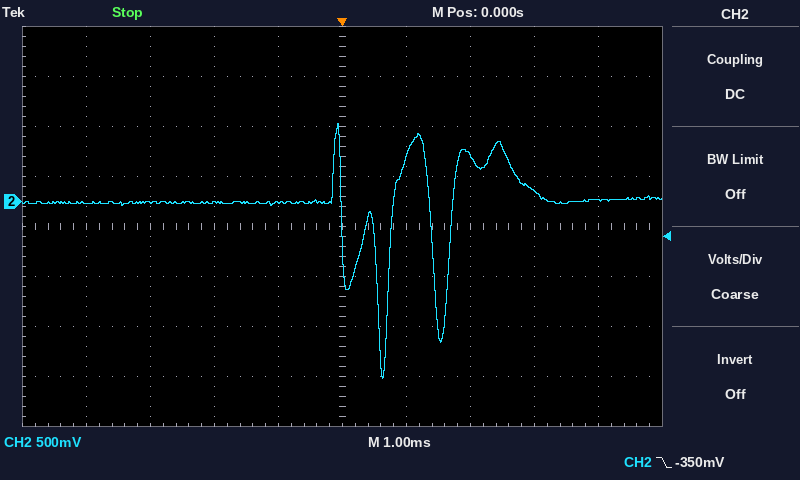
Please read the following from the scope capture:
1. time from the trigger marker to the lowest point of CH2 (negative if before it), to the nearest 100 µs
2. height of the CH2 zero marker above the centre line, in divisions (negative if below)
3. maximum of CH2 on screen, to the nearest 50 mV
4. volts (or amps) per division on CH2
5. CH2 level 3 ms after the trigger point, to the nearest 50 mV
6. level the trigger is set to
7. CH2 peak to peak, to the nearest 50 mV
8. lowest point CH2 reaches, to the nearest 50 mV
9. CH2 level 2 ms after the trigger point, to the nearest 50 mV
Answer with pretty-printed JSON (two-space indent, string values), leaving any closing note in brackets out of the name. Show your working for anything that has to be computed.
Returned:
{
  "time from the trigger marker to the lowest point of CH2 (negative if before it), to the nearest 100 µs": "+600 µs",
  "height of the CH2 zero marker above the centre line, in divisions": "+0.5 div",
  "maximum of CH2 on screen, to the nearest 50 mV": "800 mV",
  "volts (or amps) per division on CH2": "500 mV",
  "CH2 level 3 ms after the trigger point, to the nearest 50 mV": "100 mV",
  "level the trigger is set to": "-350 mV",
  "CH2 peak to peak, to the nearest 50 mV": "800 mV − (-1.75 V) = 2.55 V",
  "lowest point CH2 reaches, to the nearest 50 mV": "-1.75 V",
  "CH2 level 2 ms after the trigger point, to the nearest 50 mV": "450 mV"
}
